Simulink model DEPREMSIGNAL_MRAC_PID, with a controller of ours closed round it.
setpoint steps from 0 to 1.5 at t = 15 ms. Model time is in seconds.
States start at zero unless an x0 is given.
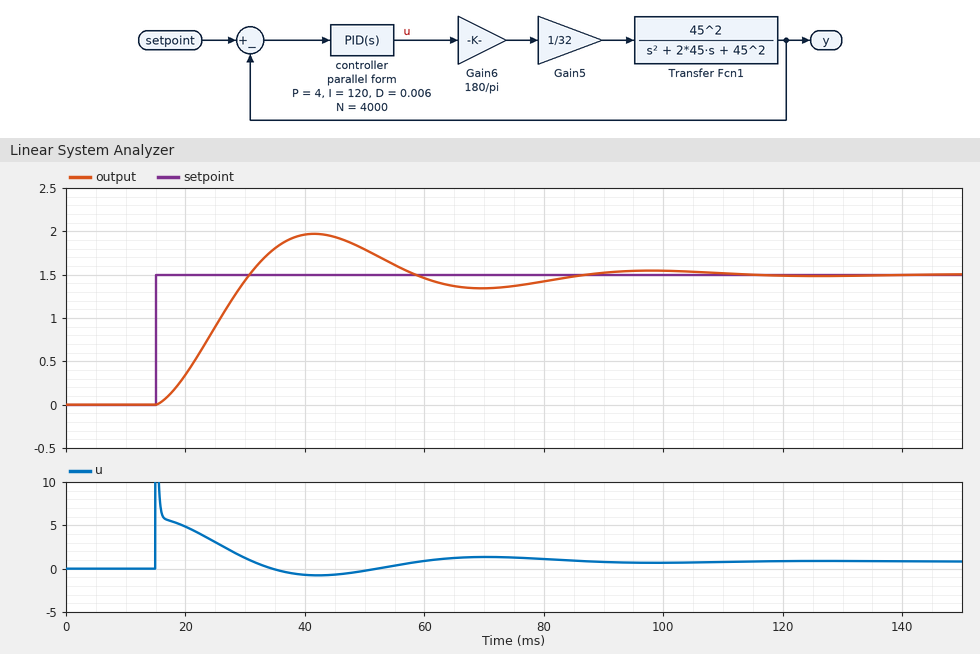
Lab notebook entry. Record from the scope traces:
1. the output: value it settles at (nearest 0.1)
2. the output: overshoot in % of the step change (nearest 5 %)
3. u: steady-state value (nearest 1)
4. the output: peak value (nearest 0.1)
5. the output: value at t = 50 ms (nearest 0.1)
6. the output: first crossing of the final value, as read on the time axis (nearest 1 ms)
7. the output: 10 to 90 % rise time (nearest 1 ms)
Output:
1.5
30 %
1
2.0
1.8
31 ms
11 ms
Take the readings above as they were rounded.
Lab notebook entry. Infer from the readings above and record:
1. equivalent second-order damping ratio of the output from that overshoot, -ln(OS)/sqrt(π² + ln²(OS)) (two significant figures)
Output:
0.36
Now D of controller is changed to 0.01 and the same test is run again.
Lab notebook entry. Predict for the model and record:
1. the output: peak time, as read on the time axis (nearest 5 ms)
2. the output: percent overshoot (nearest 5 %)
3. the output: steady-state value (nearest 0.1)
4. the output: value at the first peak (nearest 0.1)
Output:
40 ms
25 %
1.5
1.9
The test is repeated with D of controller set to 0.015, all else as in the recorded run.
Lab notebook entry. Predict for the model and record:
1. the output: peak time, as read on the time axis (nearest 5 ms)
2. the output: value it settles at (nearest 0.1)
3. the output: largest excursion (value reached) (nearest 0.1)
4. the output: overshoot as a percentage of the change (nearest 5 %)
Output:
40 ms
1.5
1.8
20 %
